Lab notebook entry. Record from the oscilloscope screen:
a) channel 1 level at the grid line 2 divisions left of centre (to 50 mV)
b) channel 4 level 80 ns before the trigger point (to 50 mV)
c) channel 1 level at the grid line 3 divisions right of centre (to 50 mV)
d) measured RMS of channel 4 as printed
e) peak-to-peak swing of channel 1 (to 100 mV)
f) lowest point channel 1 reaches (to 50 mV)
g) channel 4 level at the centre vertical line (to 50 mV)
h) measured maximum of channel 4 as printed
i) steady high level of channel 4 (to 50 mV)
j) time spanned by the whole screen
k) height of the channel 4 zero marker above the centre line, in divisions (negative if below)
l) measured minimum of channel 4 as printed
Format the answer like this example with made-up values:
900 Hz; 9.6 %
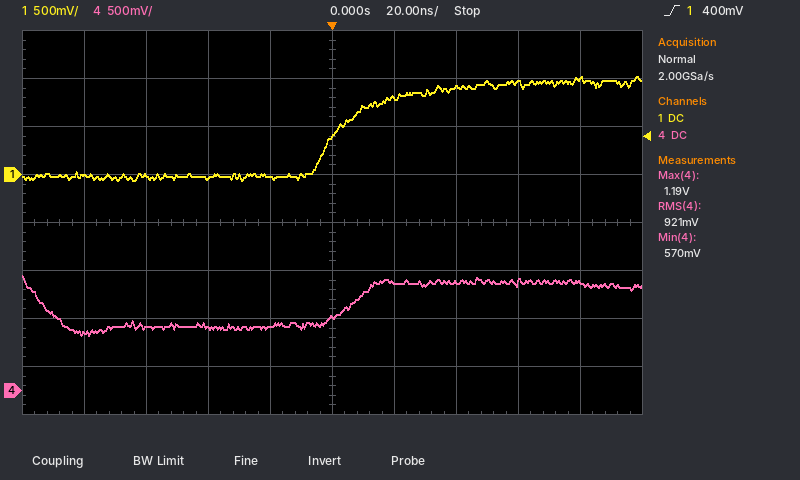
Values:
-50 mV; 600 mV; 950 mV; 921 mV; 1.10 V; -50 mV; 750 mV; 1.19 V; 1.10 V; 200 ns; -3.5 div; 570 mV
